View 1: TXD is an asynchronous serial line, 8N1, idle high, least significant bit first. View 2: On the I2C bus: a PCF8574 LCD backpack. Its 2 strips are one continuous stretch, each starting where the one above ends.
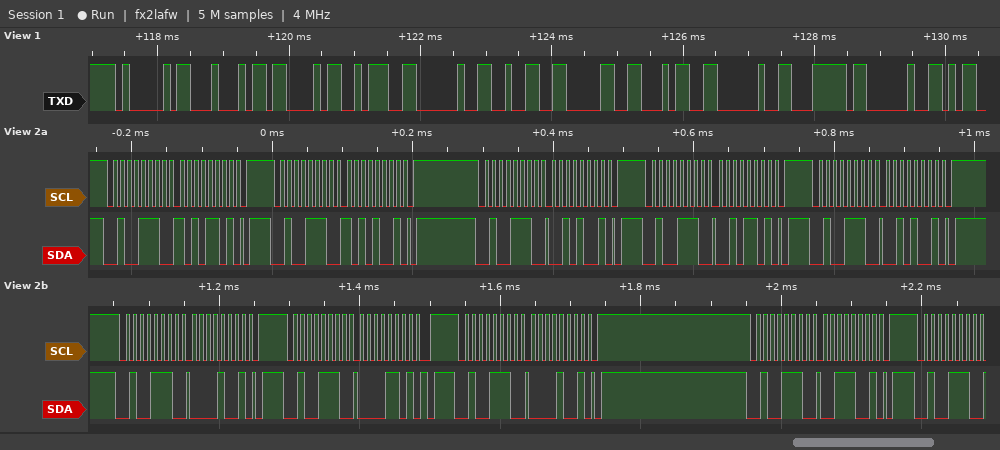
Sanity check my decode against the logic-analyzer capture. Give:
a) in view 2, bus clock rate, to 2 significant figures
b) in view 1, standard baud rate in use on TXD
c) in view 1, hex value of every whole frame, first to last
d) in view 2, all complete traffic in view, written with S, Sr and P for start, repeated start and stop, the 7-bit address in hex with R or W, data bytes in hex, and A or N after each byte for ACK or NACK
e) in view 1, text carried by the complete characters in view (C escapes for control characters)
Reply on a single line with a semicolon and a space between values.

100 kHz; 9600 baud; 41 44 43 3A 20 32 30 34 20 7C 20; S 27W A AD A P S 27W A A9 A P S 27W A 29 A P S 27W A 2D A P S 27W A 29 A P S 27W A 09 A P S 27W A 0D A P S 27W A 09 A P S 27W A 39 A P S 27W A; "ADC: 204 | "
